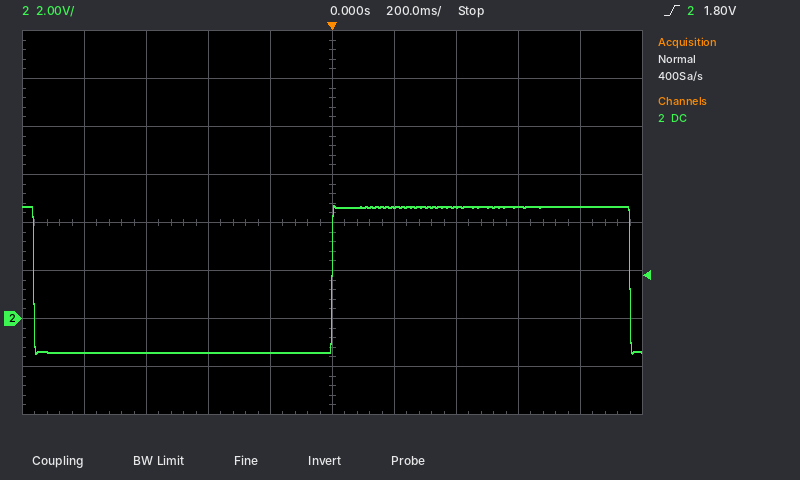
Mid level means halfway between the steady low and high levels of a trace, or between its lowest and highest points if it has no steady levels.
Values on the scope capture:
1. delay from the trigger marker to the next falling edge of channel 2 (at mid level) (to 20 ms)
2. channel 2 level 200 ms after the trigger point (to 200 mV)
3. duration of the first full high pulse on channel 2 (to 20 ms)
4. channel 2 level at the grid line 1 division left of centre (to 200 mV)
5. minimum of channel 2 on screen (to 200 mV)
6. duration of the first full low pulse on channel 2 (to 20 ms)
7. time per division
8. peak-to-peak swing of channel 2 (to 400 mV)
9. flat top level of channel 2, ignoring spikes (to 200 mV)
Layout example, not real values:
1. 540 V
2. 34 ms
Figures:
1. 960 ms
2. 4.6 V
3. 960 ms
4. -1.4 V
5. -1.4 V
6. 960 ms
7. 200 ms
8. 6.0 V
9. 4.6 V
